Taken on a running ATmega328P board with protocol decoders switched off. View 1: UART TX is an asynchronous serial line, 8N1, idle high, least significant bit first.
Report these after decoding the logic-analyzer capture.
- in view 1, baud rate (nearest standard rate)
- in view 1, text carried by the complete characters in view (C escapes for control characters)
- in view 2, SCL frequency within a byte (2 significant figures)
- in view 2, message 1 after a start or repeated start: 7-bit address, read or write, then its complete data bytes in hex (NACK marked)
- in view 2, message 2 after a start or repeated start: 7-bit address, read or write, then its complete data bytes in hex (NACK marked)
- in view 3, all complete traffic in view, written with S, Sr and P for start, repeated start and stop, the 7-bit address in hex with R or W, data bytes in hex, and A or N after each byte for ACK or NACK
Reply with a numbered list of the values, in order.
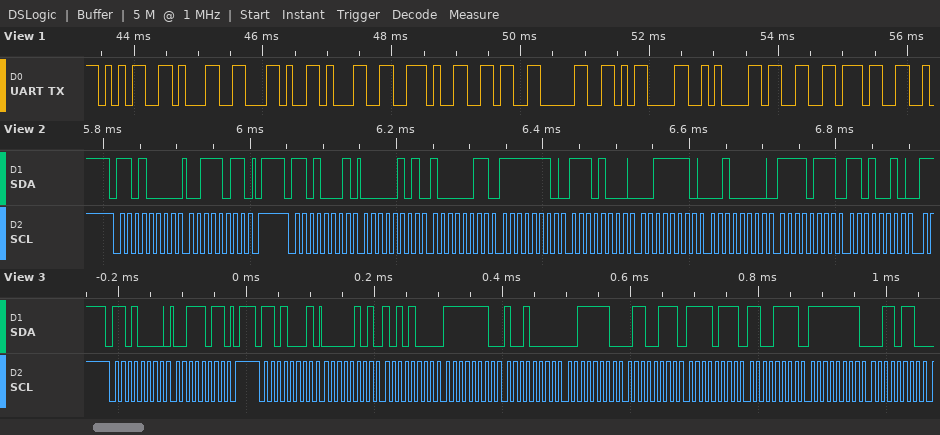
1. 9600 baud
2. "51,1.60\r\n37"
3. 100 kHz
4. 0x68 write: 3B
5. 0x68 read: 05 83 FE E8 3E 20 F7 D2
6. S 68W A 3B A P S 68R A 05 A A8 A FE A 90 A 3E A 67 A F7 A CF A FF A 36 A
